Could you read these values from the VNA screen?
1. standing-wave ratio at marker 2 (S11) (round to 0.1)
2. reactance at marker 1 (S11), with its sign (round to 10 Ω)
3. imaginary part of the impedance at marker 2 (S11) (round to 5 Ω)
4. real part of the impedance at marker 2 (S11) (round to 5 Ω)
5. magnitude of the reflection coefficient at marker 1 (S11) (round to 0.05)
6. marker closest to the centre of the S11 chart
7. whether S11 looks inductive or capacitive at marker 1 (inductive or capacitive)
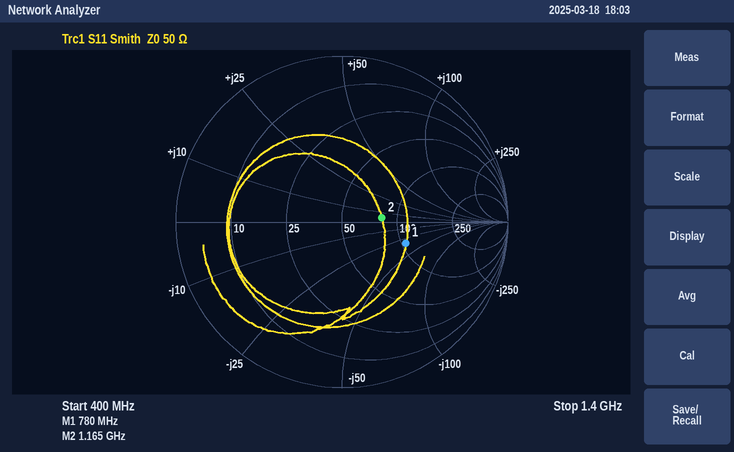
1.6
-30 Ω
+5 Ω
80 Ω
0.40
marker 2
capacitive
